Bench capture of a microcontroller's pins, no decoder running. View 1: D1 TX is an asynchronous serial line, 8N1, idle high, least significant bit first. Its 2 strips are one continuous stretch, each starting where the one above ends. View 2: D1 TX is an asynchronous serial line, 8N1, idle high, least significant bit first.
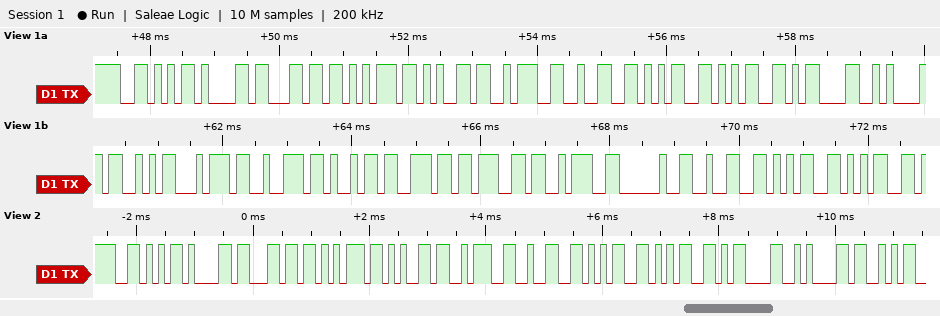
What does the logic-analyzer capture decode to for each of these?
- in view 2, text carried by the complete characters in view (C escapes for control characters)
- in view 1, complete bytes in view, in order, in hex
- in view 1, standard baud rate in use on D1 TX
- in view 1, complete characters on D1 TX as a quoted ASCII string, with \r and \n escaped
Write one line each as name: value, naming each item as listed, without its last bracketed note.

in view 2, text carried by the complete characters in view: "Value:255\r\nS"
in view 1, complete bytes in view, in order, in hex: 56 61 6C 75 65 3A 32 35 35 0D 0A 53 74 72 69 6E 67 3A 20 32 35 35
in view 1, standard baud rate in use on D1 TX: 9600 baud
in view 1, complete characters on D1 TX as a quoted ASCII string, with \r and \n escaped: "Value:255\r\nString: 255"
